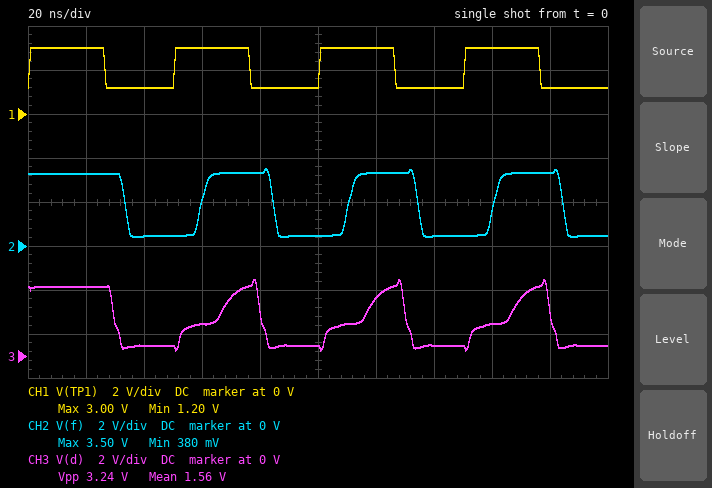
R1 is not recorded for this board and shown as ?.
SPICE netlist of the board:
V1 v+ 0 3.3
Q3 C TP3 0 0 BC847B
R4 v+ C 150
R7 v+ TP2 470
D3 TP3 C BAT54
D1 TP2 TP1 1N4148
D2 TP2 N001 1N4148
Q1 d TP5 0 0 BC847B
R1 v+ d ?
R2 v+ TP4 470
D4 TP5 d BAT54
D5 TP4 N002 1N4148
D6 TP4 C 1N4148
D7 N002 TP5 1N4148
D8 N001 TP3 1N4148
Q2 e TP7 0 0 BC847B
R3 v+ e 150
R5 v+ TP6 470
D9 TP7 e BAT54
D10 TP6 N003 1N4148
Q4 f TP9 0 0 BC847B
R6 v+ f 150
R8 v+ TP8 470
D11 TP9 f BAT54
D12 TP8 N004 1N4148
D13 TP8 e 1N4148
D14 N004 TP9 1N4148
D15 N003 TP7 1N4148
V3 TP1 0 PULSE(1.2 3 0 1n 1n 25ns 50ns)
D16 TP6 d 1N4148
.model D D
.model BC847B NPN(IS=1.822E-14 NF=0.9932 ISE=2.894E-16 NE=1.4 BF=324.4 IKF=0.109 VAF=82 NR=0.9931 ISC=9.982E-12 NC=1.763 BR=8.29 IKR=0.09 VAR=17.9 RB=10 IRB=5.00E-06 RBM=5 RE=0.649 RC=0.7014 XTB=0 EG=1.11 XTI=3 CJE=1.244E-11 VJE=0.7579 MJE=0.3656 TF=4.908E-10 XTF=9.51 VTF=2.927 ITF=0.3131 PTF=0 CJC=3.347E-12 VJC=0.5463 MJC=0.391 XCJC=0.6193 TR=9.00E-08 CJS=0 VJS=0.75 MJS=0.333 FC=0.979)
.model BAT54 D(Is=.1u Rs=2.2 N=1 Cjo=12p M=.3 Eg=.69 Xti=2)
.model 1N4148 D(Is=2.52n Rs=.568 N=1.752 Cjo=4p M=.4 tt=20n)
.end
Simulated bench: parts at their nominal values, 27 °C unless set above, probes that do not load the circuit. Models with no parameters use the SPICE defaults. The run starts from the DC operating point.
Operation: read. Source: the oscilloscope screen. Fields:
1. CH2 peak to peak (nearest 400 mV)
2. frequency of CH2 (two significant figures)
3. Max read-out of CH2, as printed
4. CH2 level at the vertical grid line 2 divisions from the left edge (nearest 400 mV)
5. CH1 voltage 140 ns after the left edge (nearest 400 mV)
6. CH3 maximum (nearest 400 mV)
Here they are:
3.2 V
20 MHz
3.50 V
400 mV
1.2 V
3.6 V
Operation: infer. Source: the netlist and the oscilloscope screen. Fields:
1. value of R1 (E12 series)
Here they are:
390 Ω
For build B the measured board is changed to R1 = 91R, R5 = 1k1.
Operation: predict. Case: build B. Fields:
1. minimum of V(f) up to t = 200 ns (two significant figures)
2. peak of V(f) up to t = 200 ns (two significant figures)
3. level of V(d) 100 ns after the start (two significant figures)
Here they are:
420 mV
3.6 V
490 mV
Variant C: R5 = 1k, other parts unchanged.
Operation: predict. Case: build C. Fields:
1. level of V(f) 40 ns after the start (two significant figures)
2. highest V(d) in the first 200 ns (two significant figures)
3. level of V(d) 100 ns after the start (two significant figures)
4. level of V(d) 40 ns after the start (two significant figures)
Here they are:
420 mV
3.6 V
440 mV
440 mV
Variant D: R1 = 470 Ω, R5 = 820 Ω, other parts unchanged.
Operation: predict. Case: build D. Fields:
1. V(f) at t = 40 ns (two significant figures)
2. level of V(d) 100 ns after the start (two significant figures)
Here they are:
450 mV
440 mV
